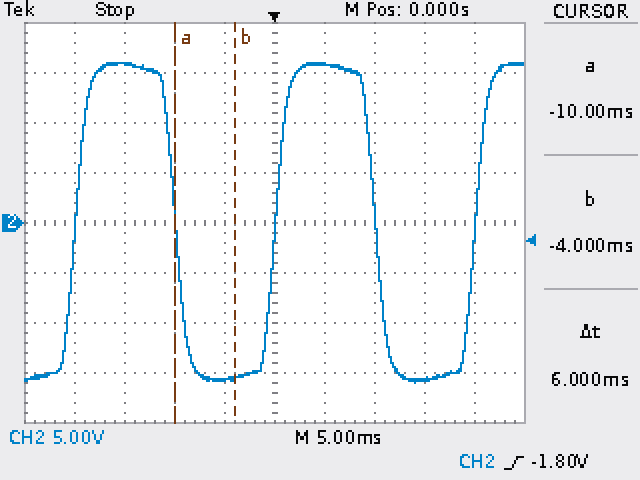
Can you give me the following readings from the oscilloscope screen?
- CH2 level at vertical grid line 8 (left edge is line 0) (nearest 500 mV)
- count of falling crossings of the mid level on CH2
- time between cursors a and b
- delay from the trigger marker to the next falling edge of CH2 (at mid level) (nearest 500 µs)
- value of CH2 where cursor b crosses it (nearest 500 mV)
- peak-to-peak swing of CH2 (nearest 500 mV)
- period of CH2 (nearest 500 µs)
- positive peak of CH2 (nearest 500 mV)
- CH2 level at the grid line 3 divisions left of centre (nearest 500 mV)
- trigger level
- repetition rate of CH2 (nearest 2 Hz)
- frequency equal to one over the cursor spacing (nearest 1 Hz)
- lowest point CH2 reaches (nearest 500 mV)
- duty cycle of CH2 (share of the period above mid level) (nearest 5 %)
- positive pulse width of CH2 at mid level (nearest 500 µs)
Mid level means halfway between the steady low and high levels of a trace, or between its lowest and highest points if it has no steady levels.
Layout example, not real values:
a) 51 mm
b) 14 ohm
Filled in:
a) -15.5 V
b) 2
c) 6 ms
d) 10.0 ms
e) -15.5 V
f) 32.0 V
g) 20.0 ms
h) 16.0 V
i) 16.0 V
j) -1.80 V
k) 50 Hz
l) 167 Hz
m) -16.0 V
n) 50 %
o) 10.0 ms
